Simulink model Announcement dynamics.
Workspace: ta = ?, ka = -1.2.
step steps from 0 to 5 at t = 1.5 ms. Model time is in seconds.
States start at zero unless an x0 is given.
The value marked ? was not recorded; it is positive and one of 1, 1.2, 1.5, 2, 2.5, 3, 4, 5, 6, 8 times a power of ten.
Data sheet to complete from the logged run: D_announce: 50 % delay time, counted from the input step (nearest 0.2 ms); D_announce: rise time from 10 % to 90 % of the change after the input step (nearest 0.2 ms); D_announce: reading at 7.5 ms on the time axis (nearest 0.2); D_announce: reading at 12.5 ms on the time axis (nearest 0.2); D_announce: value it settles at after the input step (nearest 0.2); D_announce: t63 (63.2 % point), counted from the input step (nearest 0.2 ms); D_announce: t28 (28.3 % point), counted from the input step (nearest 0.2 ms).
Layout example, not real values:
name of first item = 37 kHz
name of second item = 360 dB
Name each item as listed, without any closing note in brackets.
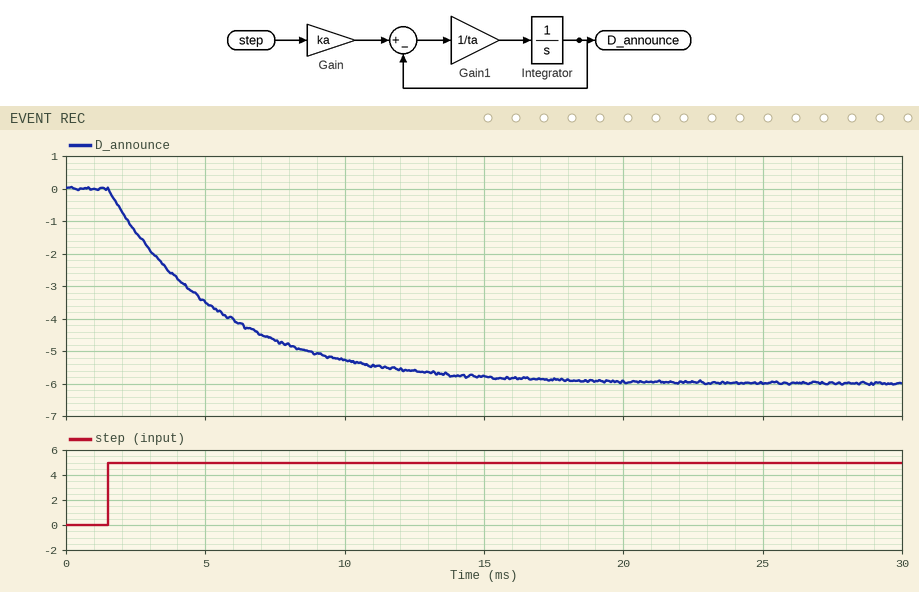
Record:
D_announce: 50 % delay time, counted from the input step = 2.8 ms
D_announce: rise time from 10 % to 90 % of the change after the input step = 8.8 ms
D_announce: reading at 7.5 ms on the time axis = -4.6
D_announce: reading at 12.5 ms on the time axis = -5.6
D_announce: value it settles at after the input step = -6.0
D_announce: t63 (63.2 % point), counted from the input step = 4.0 ms
D_announce: t28 (28.3 % point), counted from the input step = 1.4 ms
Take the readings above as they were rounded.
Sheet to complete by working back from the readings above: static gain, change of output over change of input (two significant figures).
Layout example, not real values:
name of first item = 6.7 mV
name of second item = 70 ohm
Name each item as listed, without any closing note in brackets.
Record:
static gain, change of output over change of input = -1.2
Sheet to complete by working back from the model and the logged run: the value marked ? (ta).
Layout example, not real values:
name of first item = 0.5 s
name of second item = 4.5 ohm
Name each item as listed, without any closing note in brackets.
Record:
the value marked ? = 0.004
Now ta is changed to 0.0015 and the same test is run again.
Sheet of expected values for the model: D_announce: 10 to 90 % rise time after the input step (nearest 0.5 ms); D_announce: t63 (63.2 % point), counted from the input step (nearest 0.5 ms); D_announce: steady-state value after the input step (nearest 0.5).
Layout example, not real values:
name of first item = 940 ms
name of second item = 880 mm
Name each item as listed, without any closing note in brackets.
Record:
D_announce: 10 to 90 % rise time after the input step = 3.5 ms
D_announce: t63 (63.2 % point), counted from the input step = 1.5 ms
D_announce: steady-state value after the input step = -6.0
